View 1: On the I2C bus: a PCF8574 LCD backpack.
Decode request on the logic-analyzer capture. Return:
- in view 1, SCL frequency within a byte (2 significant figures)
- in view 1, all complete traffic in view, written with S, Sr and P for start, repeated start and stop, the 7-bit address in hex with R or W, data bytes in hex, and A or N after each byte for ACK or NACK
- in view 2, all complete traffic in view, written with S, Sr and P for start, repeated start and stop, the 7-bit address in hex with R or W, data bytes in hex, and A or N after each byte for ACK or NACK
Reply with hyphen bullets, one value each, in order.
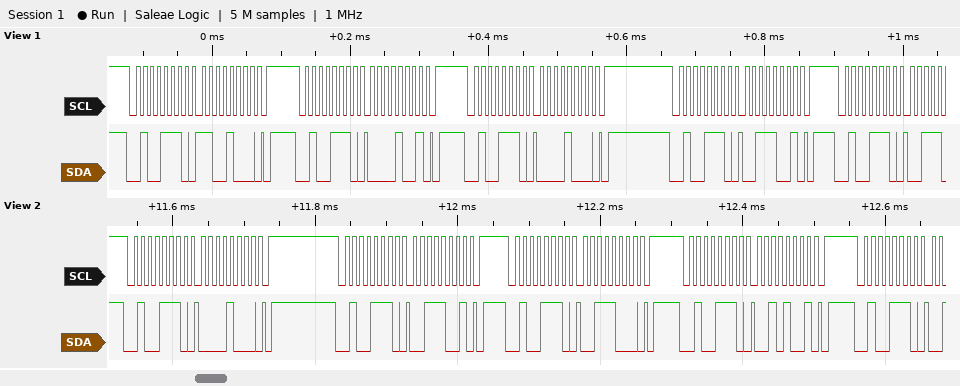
- 100 kHz
- S 27W A C8 A P S 27W A 09 A P S 27W A 08 A P S 27W A 39 A P S 27W A
- S 27W A 08 A P S 27W A 39 A P S 27W A 38 A P S 27W A 29 A P S 27W A
